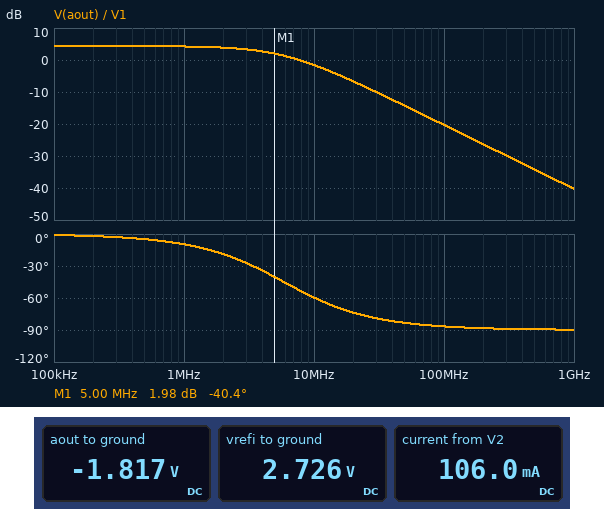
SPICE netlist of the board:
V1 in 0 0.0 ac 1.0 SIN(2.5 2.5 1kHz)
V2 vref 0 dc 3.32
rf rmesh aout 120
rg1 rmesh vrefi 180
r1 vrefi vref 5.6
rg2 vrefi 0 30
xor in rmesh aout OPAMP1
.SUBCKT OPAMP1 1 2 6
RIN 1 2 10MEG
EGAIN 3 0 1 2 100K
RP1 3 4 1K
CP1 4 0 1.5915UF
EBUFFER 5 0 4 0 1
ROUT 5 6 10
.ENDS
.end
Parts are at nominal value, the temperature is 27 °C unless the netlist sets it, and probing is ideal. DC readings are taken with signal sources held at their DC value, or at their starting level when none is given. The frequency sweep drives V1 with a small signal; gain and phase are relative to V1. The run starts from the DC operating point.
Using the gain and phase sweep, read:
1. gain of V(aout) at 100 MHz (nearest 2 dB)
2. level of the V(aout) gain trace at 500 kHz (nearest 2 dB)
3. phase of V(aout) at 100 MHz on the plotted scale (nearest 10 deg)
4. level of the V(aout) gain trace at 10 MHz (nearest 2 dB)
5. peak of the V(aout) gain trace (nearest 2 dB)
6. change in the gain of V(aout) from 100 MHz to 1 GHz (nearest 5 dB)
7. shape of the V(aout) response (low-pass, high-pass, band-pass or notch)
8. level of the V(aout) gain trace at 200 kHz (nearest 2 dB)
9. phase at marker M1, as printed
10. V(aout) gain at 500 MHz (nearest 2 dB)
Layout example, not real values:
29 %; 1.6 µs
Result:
-20 dB; 4 dB; -90 deg; -2 dB; 4 dB; -20 dB; low-pass; 4 dB; -40.4 deg; -34 dB
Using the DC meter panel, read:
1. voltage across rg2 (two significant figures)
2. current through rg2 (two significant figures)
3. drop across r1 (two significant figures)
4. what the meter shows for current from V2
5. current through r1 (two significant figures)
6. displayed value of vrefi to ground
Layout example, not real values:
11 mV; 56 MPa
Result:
2.7 V; 91 mA; 590 mV; 106.0 mA; 110 mA; 2.726 V
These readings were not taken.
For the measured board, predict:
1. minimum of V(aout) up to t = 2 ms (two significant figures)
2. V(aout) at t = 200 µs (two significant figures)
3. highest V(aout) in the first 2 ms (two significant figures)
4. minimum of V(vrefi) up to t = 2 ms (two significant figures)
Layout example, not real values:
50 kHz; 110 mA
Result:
-1.8 V; 6.2 V; 6.4 V; 2.7 V
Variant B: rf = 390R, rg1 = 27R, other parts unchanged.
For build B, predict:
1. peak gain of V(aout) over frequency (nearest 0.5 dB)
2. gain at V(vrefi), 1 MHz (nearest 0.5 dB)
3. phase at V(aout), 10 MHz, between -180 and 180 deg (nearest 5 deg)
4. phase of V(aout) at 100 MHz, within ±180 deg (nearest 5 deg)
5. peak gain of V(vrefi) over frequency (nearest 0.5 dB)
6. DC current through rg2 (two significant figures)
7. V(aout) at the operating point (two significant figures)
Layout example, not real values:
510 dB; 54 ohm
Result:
22.5 dB; -21.0 dB; -85 deg; -90 deg; -16.5 dB; 79 mA; -34 V
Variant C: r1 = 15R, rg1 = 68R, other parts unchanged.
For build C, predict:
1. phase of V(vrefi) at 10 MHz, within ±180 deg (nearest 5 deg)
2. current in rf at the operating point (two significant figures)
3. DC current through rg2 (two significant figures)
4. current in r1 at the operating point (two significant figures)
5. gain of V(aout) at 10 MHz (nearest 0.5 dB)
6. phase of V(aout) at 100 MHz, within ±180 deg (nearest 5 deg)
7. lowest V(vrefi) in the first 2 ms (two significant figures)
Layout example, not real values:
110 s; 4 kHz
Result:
-70 deg; 28 mA; 64 mA; 93 mA; -1.0 dB; -90 deg; 1.9 V
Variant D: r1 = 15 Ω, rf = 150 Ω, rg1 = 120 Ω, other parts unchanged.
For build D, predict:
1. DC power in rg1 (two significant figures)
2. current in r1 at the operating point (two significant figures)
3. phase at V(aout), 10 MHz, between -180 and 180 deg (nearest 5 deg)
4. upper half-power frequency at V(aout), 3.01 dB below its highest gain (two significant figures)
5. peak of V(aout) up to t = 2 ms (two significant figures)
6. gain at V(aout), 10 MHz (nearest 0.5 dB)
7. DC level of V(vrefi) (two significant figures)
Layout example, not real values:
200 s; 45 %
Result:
35 mW; 85 mA; -65 deg; 4.5 MHz; 8.2 V; -1.0 dB; 2.0 V
